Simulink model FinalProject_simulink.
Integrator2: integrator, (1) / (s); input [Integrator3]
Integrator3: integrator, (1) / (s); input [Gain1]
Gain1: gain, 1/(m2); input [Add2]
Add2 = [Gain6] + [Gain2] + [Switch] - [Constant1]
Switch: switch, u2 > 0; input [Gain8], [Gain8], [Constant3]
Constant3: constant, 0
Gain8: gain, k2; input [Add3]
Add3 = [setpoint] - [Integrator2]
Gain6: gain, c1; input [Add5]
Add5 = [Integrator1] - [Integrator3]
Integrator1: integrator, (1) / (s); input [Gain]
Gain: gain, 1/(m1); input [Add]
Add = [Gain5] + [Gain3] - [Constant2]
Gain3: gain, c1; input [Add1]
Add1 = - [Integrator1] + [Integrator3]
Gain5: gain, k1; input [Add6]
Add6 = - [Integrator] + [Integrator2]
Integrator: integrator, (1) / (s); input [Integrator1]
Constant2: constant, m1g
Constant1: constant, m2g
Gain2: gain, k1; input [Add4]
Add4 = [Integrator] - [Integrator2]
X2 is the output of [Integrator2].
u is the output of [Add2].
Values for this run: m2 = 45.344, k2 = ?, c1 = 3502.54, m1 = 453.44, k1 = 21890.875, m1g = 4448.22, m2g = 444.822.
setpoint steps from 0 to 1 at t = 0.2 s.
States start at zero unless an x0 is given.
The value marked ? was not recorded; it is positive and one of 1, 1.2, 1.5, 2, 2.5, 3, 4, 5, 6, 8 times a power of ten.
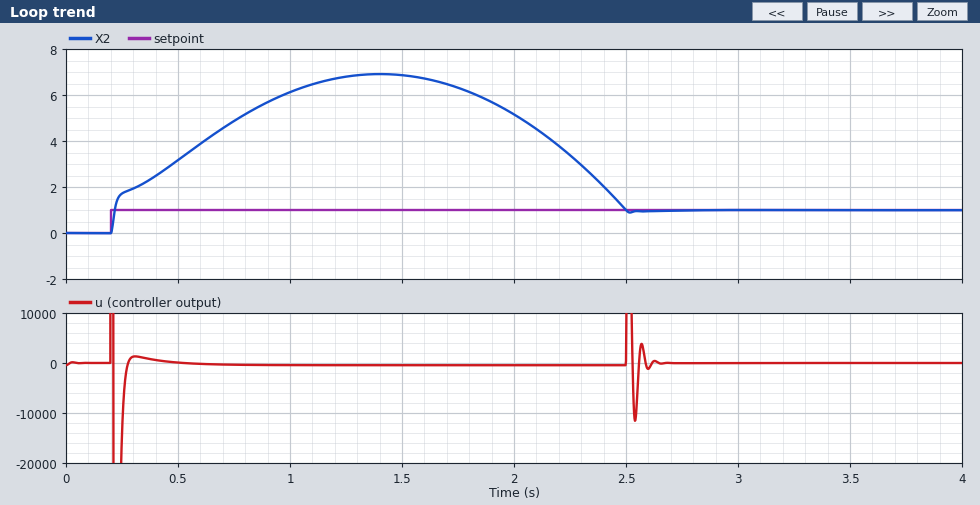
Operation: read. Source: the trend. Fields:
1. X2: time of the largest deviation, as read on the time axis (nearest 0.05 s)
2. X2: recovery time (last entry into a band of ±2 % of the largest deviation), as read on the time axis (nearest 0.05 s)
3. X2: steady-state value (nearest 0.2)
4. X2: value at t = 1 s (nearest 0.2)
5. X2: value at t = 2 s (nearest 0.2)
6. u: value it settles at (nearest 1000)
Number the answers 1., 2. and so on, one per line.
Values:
1. 1.40 s
2. 2.50 s
3. 1.0
4. 6.2
5. 5.2
6. 0
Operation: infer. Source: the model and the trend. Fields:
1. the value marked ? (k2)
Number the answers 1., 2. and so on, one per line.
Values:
1. 600000
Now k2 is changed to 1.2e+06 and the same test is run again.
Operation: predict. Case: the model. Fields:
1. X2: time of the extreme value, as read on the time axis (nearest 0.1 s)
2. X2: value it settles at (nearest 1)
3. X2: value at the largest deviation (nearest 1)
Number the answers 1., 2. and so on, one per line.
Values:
1. 1.8 s
2. 1
3. 13
